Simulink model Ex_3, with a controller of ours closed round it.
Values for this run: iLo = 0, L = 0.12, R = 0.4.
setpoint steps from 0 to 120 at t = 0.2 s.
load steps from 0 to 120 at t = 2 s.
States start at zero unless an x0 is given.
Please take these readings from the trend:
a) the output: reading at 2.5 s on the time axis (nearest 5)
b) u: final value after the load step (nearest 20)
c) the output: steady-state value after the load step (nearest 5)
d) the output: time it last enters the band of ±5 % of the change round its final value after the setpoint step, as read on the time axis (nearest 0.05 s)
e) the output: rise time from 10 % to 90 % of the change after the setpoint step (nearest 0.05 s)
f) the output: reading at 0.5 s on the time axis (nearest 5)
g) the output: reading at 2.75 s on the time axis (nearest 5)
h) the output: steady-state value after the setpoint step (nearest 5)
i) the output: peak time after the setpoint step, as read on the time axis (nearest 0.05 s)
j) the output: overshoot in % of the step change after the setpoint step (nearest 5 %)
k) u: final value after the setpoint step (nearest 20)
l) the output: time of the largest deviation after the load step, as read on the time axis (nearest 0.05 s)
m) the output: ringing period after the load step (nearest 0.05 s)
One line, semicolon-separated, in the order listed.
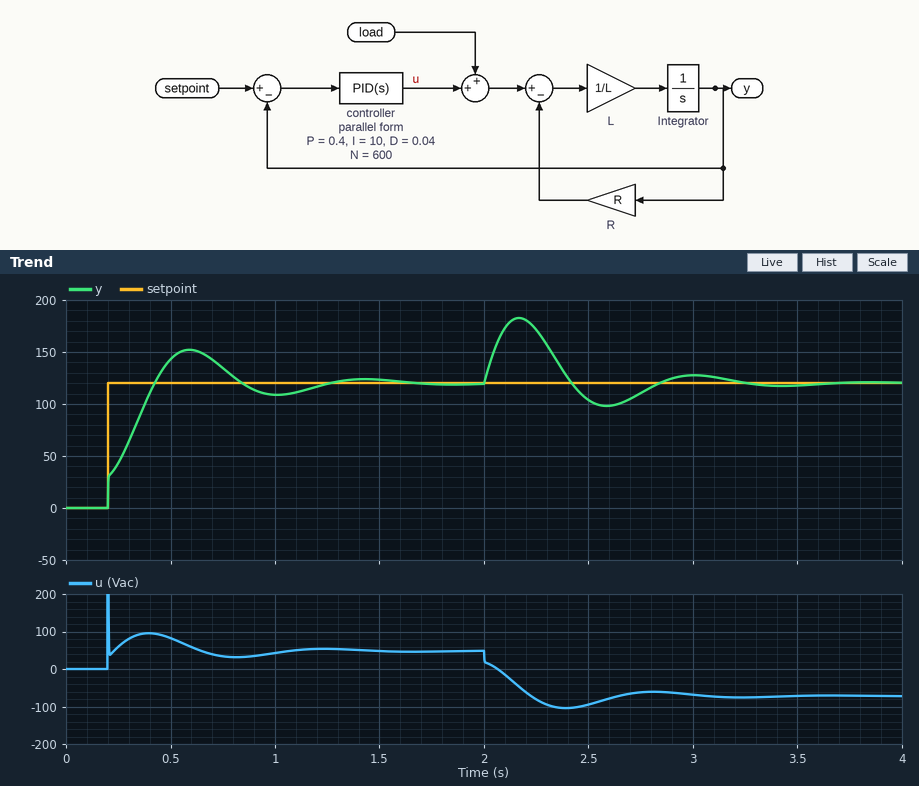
105; -80; 120; 1.15 s; 0.20 s; 145; 110; 120; 0.60 s; 25 %; 40; 2.15 s; 0.85 s
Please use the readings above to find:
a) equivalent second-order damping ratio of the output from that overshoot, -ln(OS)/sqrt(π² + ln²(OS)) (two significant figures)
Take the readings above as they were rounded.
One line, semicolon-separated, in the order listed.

0.40
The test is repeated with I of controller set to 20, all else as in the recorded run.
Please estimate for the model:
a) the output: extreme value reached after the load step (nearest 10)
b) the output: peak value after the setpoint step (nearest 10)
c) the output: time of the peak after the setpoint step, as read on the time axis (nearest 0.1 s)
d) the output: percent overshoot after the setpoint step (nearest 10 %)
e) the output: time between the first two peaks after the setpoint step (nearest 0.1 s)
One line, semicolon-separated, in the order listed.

170; 160; 0.5 s; 40 %; 0.6 s
